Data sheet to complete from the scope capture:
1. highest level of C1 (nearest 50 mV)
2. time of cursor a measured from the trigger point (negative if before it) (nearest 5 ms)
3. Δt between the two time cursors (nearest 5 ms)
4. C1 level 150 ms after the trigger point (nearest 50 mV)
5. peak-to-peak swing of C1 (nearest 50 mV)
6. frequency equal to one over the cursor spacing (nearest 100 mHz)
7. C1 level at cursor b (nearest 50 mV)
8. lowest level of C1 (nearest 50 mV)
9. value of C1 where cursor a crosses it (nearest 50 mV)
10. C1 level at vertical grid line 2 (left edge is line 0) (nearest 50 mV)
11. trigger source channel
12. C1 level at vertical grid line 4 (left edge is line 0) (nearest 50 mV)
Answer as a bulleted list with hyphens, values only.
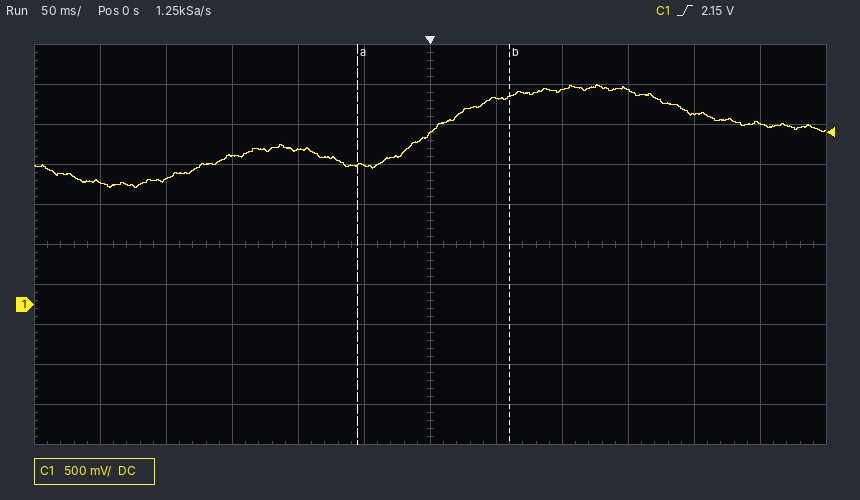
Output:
- 2.75 V
- -55 ms
- 115 ms
- 2.70 V
- 1.30 V
- 8.7 Hz
- 2.60 V
- 1.45 V
- 1.75 V
- 1.55 V
- C1
- 1.95 V
